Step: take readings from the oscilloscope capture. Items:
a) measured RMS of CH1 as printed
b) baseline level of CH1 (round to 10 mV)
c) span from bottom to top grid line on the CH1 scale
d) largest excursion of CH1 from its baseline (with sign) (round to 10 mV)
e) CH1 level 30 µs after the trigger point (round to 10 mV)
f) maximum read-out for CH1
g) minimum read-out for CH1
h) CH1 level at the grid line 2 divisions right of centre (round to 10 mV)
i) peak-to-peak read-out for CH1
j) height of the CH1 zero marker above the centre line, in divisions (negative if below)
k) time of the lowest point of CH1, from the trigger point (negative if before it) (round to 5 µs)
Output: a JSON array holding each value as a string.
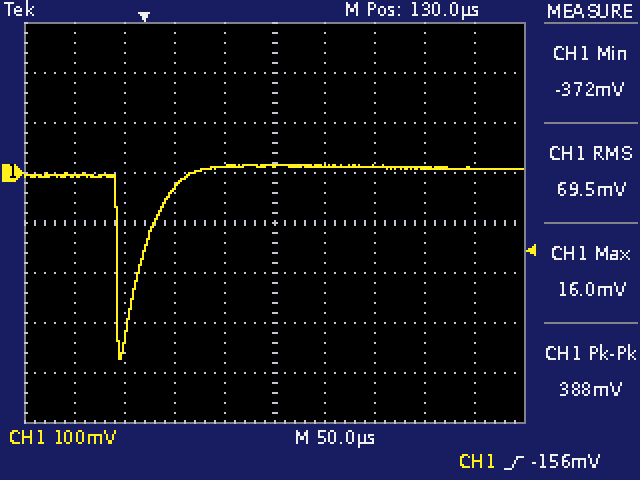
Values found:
["69.5 mV", "10 mV", "800 mV", "-380 mV", "-30 mV", "16.0 mV", "-372 mV", "10 mV", "388 mV", "+1.0 div", "-25 µs"]
